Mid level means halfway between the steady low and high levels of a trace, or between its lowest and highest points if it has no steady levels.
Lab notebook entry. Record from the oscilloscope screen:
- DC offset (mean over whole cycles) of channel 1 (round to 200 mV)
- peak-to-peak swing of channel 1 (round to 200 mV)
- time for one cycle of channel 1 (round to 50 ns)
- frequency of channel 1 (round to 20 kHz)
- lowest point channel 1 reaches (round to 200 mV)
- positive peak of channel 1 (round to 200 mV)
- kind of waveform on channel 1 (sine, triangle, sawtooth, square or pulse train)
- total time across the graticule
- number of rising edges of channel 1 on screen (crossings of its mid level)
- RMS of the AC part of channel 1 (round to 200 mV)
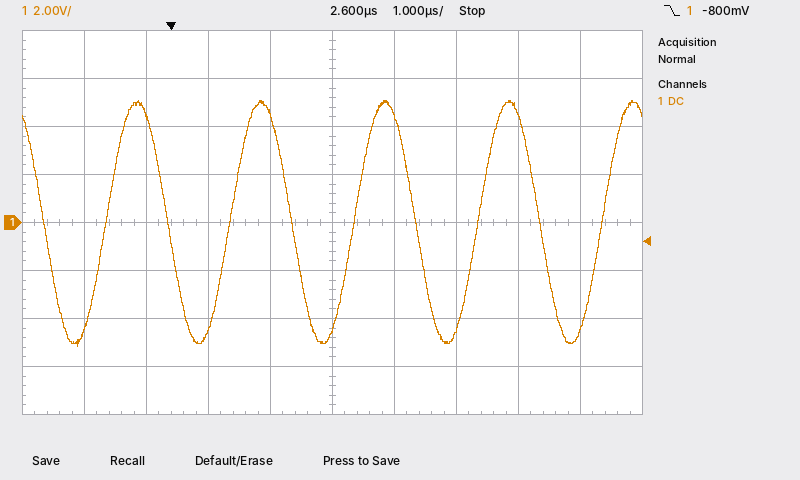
0.0 V
10.2 V
2.00 µs
500 kHz
-5.2 V
5.0 V
sine
10 µs
5
3.6 V
